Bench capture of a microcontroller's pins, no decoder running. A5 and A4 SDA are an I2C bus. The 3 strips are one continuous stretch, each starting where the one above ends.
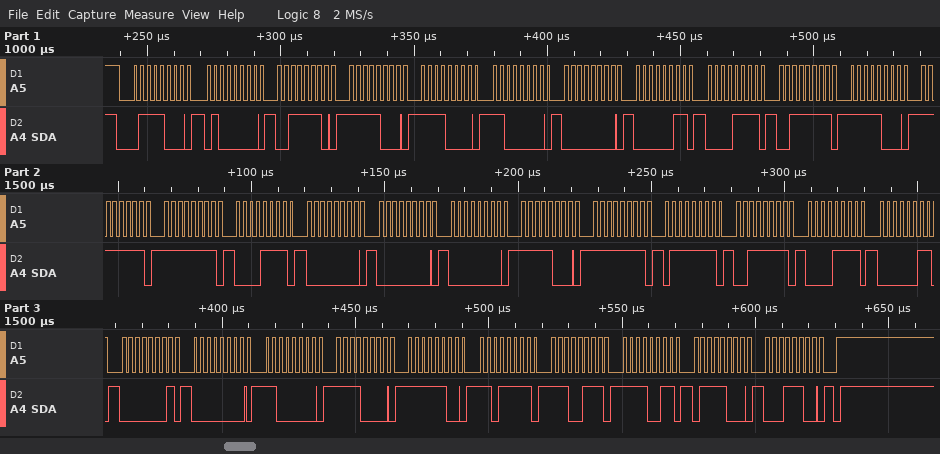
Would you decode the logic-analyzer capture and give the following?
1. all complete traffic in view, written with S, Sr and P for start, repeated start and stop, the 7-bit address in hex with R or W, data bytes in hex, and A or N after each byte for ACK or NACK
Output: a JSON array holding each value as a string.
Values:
["S 3CW A 40 A 3E A F8 A F0 A C0 A 00 A 03 A 0F A 3F A F8 A FF A FF A 0F A 00 A 00 A 00 A F8 A FF A 7F A 3F A 0F A 03 A 01 A 00 A C0 A F0 A FC A DF A E7 A F3 A 78 A 1C A P"]
